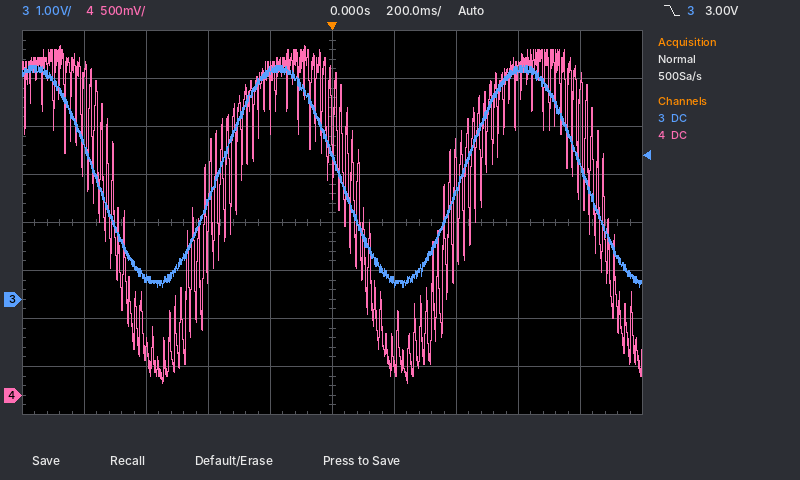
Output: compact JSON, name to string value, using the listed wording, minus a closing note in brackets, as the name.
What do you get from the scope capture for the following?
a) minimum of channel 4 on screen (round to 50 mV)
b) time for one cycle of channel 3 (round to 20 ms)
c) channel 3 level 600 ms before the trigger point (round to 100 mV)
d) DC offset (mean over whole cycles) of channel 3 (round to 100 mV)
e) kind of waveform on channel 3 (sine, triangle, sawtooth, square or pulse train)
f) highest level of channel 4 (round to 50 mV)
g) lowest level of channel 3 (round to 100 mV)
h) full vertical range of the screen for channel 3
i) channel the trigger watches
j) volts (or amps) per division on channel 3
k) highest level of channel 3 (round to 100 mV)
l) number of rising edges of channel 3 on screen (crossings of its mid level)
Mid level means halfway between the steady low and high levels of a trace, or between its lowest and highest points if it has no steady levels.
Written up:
{"minimum of channel 4 on screen": "100 mV", "time for one cycle of channel 3": "780 ms", "channel 3 level 600 ms before the trigger point": "400 mV", "DC offset (mean over whole cycles) of channel 3": "2.6 V", "kind of waveform on channel 3": "sine", "highest level of channel 4": "3.65 V", "lowest level of channel 3": "200 mV", "full vertical range of the screen for channel 3": "8 V", "channel the trigger watches": "channel 3", "volts (or amps) per division on channel 3": "1 V", "highest level of channel 3": "4.9 V", "number of rising edges of channel 3 on screen": "2"}
